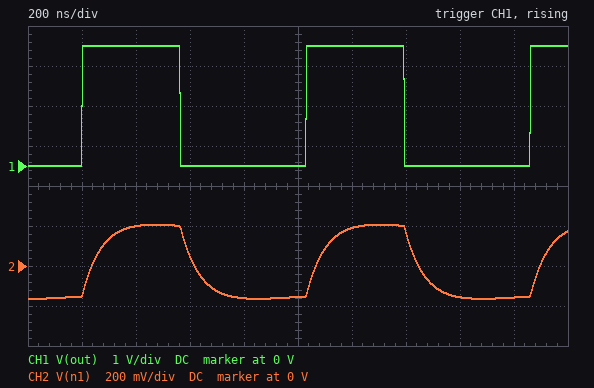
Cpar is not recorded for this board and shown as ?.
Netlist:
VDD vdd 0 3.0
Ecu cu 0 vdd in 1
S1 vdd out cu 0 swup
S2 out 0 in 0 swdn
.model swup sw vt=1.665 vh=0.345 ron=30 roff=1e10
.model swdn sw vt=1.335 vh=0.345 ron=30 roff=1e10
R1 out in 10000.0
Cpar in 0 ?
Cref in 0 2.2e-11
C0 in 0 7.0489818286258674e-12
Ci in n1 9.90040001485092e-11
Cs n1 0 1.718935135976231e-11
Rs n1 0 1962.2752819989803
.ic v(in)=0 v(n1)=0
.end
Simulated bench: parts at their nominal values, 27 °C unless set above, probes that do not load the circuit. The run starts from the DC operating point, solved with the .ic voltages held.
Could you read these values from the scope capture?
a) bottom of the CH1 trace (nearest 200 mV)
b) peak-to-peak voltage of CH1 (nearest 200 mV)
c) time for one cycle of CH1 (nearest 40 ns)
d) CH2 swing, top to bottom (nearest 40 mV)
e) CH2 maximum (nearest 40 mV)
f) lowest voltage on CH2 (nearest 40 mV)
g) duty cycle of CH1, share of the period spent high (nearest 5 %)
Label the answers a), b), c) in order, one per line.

a) 0 V
b) 3.0 V
c) 840 ns
d) 360 mV
e) 200 mV
f) -160 mV
g) 45 %
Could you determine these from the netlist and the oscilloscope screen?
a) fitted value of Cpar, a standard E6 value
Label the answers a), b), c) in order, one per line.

a) 4.7 pF
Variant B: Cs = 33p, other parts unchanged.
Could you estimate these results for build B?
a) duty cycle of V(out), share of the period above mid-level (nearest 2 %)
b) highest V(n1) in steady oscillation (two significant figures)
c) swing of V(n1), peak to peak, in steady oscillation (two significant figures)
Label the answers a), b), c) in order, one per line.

a) 44 %
b) 200 mV
c) 350 mV
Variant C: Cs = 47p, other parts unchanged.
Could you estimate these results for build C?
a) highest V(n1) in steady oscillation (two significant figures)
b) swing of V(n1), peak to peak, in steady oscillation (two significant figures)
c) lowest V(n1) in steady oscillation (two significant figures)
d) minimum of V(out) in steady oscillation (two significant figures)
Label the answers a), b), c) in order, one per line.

a) 190 mV
b) 340 mV
c) -150 mV
d) 3.0 mV
